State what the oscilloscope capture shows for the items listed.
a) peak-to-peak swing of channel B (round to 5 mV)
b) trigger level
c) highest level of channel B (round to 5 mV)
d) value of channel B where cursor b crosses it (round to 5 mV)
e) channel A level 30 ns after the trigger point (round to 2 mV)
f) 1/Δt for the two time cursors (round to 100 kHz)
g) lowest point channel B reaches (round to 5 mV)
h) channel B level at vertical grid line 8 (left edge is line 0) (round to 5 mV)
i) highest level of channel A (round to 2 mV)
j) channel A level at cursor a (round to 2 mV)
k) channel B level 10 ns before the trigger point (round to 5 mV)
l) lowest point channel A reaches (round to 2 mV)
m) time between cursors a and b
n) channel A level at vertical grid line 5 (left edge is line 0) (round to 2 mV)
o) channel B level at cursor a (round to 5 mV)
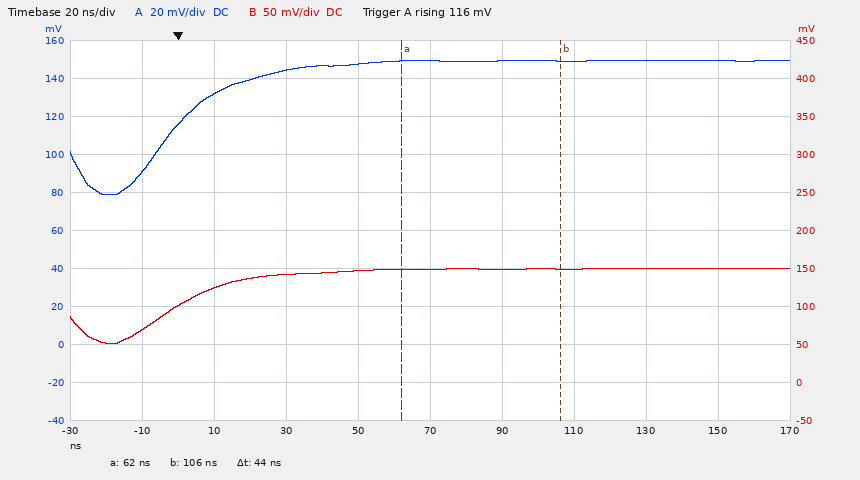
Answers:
100 mV
116 mV
150 mV
150 mV
144 mV
22.7 MHz
50 mV
150 mV
150 mV
150 mV
70 mV
78 mV
44 ns
150 mV
150 mV
